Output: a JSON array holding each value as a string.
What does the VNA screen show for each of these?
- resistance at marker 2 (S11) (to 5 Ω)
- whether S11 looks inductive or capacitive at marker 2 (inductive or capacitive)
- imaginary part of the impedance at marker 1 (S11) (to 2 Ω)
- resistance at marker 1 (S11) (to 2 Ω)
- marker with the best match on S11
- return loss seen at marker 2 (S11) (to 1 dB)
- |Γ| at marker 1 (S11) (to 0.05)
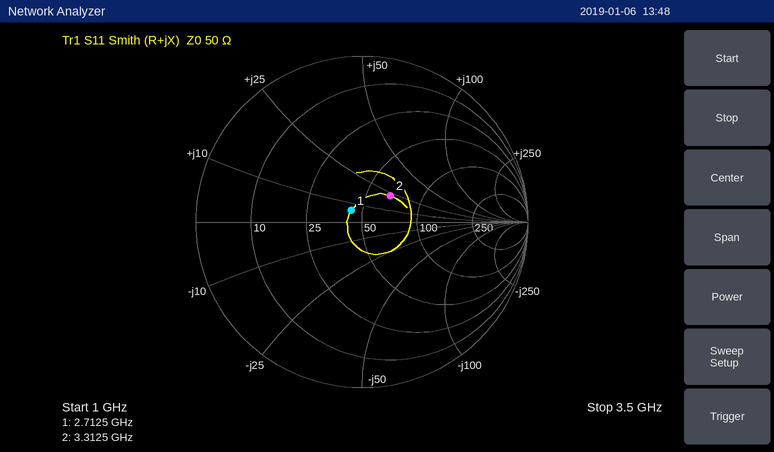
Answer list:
["65 Ω", "inductive", "+6 Ω", "44 Ω", "marker 1", "13 dB", "0.10"]
